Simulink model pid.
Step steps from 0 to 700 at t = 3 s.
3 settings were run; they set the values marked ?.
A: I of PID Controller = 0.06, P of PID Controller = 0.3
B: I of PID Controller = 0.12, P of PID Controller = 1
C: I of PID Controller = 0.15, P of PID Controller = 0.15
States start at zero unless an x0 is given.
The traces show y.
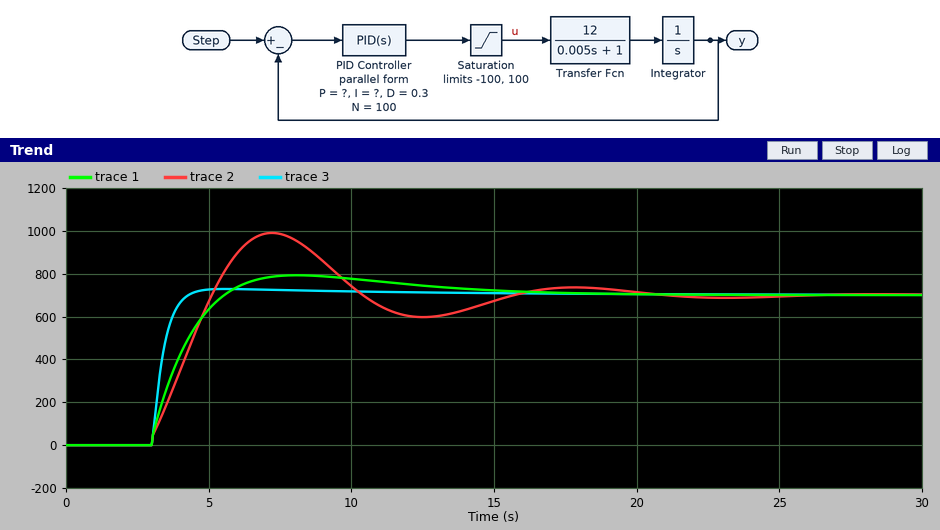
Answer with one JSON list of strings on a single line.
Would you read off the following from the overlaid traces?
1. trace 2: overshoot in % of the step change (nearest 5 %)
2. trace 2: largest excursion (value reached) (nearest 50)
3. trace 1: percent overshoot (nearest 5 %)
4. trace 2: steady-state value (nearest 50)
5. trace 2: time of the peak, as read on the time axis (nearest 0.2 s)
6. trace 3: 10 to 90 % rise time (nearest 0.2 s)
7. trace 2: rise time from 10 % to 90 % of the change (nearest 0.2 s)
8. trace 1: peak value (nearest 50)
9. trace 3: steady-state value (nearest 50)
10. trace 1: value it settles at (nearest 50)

["40 %", "1000", "15 %", "700", "7.2 s", "0.8 s", "1.8 s", "800", "700", "700"]
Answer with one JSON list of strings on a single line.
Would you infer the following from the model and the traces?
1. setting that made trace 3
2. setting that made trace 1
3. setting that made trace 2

["B", "A", "C"]
